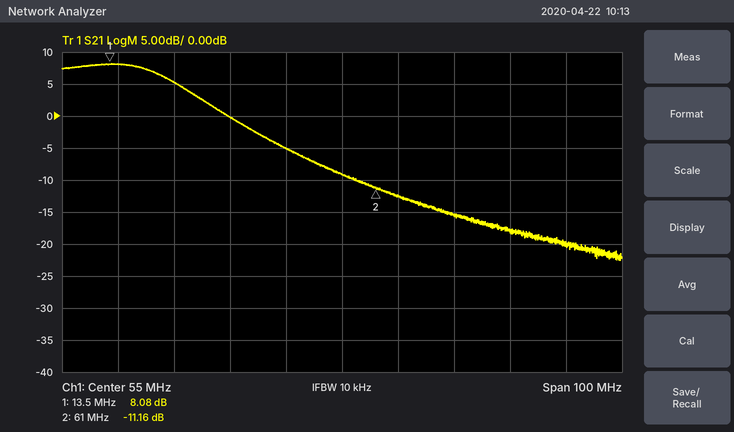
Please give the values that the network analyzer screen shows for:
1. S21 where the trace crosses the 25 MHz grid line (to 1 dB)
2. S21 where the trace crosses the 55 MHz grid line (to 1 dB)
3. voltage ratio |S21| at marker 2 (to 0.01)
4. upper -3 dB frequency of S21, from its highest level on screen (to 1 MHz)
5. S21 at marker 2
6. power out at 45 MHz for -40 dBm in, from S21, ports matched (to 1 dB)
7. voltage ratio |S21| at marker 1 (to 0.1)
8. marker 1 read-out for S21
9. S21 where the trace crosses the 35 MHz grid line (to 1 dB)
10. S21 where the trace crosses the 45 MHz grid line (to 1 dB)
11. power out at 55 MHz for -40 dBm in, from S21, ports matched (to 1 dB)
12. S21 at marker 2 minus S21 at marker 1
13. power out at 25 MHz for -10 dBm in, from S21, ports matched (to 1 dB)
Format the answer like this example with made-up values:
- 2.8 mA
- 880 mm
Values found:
- 5 dB
- -9 dB
- 0.28
- 25 MHz
- -11.16 dB
- -45 dBm
- 2.5
- 8.08 dB
- 0 dB
- -5 dB
- -49 dBm
- -19.24 dB
- -5 dBm
